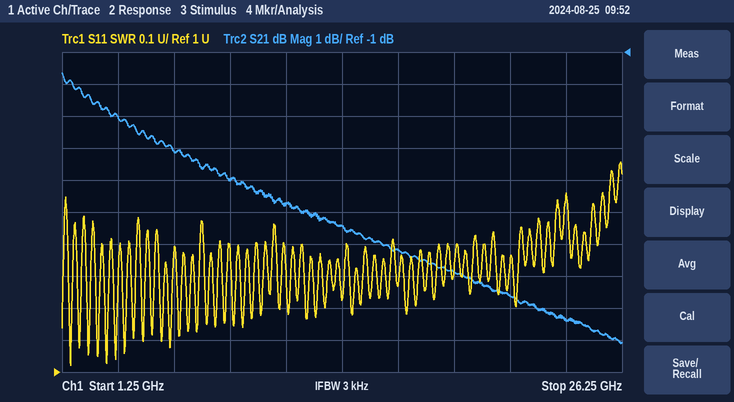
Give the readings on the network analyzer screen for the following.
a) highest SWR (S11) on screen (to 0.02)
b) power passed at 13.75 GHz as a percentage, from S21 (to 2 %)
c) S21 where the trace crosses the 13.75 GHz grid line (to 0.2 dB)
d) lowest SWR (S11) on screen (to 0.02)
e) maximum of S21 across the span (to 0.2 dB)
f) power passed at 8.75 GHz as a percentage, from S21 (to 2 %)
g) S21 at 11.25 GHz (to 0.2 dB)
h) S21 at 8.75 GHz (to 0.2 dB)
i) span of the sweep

1.66
22 %
-6.4 dB
1.02
-1.6 dB
32 %
-5.8 dB
-5.0 dB
25 GHz
